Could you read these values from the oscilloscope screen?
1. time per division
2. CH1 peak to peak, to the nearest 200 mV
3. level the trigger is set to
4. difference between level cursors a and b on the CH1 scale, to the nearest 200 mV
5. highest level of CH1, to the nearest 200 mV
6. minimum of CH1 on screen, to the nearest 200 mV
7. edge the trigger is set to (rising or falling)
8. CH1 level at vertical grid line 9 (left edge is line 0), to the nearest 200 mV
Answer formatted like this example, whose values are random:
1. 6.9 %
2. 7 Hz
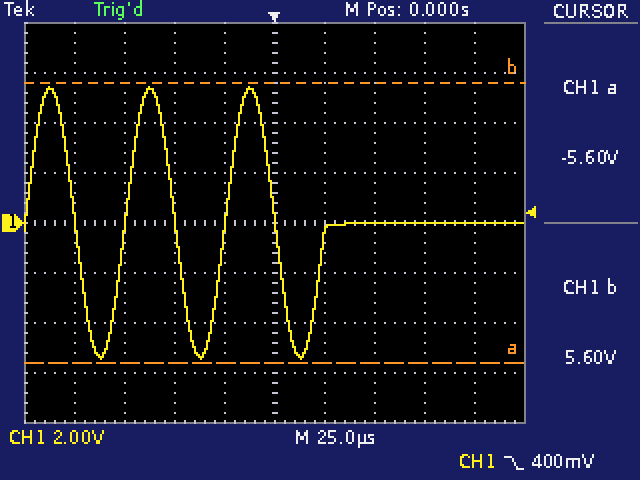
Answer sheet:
1. 25 µs
2. 10.8 V
3. 400 mV
4. 11.2 V
5. 5.4 V
6. -5.4 V
7. falling
8. 0.0 V
